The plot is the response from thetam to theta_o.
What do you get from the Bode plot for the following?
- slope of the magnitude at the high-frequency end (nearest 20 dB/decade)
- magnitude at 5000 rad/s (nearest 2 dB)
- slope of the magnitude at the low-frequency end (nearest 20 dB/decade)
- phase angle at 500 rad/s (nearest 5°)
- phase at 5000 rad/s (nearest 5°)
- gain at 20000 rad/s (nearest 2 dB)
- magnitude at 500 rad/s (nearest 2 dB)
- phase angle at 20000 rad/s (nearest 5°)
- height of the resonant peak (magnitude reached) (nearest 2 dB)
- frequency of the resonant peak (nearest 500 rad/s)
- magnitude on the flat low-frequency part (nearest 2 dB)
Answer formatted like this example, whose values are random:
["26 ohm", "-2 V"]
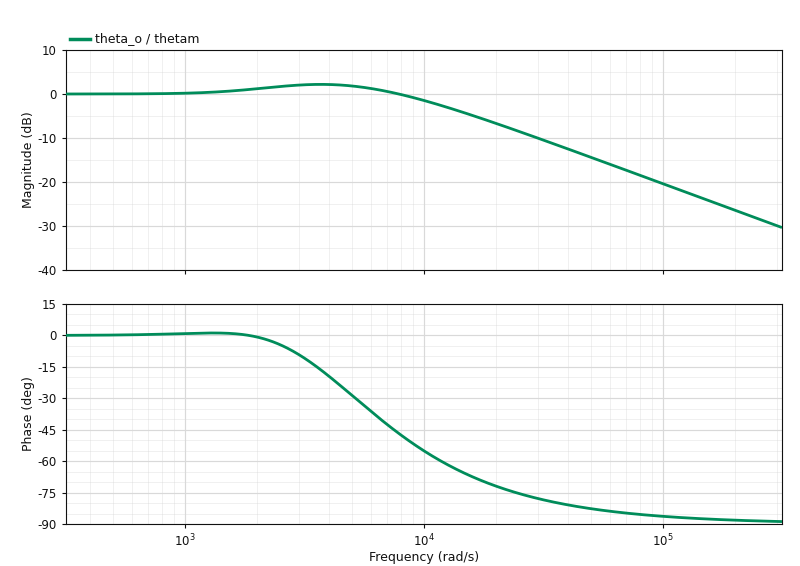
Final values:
["-20 dB/decade", "2 dB", "0 dB/decade", "0°", "-30°", "-6 dB", "0 dB", "-70°", "2 dB", "3500 rad/s", "0 dB"]
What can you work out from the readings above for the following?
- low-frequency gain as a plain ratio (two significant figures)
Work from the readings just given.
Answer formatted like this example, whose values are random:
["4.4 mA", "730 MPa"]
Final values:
["1.0"]
